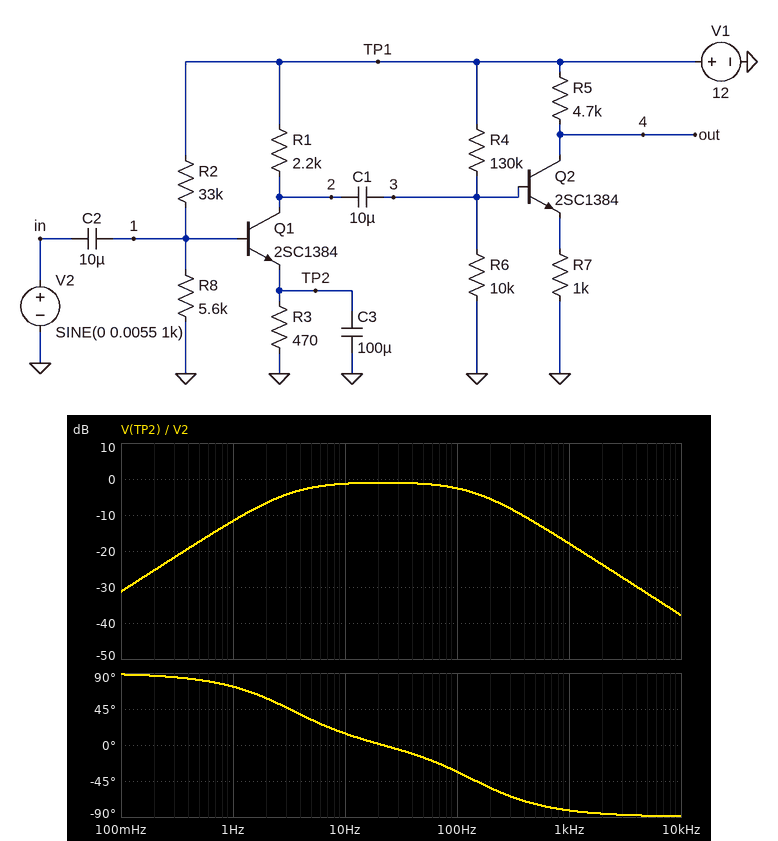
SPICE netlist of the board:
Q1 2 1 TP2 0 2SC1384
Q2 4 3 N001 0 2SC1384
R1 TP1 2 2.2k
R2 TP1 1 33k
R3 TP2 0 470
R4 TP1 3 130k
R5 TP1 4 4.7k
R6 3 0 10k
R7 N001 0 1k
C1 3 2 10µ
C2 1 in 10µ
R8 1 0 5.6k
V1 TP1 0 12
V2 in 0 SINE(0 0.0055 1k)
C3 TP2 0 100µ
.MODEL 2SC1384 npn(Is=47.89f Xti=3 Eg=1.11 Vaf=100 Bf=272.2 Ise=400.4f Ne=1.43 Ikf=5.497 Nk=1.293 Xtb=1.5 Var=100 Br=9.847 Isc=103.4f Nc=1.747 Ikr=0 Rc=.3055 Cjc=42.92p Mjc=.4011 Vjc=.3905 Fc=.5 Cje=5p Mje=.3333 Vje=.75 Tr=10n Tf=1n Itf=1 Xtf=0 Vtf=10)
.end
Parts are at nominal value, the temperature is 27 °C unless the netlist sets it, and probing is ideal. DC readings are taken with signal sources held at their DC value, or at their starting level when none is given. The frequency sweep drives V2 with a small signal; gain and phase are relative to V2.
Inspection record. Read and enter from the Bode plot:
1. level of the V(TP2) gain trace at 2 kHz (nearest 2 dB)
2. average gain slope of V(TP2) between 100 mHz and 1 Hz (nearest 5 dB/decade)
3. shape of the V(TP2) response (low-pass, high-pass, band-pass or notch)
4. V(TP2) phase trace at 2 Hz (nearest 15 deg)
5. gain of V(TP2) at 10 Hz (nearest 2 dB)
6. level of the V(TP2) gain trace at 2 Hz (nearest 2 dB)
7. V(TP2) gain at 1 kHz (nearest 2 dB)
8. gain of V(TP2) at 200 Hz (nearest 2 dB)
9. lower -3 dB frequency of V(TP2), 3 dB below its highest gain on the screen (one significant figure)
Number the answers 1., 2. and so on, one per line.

1. -24 dB
2. 20 dB/decade
3. band-pass
4. 60 deg
5. -2 dB
6. -6 dB
7. -18 dB
8. -6 dB
9. 3 Hz
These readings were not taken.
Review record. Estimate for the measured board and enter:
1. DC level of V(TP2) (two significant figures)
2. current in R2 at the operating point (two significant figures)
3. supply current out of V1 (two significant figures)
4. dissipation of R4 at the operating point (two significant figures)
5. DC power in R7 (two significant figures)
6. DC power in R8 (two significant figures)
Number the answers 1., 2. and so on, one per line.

1. 1.0 V
2. 310 µA
3. 2.8 mA
4. 960 µW
5. 63 µW
6. 490 µW
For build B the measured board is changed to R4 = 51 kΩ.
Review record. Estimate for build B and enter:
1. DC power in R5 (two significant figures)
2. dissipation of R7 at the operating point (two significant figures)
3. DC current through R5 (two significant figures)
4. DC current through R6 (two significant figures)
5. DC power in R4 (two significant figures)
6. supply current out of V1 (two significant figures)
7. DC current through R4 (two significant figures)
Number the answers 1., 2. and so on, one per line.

1. 7.2 mW
2. 1.6 mW
3. 1.2 mA
4. 190 µA
5. 2.0 mW
6. 3.9 mA
7. 200 µA
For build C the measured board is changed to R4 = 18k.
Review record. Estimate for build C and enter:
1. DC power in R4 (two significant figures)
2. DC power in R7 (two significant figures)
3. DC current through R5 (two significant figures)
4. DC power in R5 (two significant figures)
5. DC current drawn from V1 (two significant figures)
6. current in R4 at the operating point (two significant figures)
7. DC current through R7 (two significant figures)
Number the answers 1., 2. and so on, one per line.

1. 4.6 mW
2. 5.2 mW
3. 2.1 mA
4. 20 mW
5. 5.0 mA
6. 500 µA
7. 2.3 mA
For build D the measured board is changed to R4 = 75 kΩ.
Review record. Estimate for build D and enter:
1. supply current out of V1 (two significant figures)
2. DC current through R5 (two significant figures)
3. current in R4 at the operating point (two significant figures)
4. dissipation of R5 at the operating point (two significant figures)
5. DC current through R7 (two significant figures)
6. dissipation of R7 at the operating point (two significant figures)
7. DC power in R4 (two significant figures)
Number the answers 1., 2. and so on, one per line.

1. 3.3 mA
2. 730 µA
3. 140 µA
4. 2.5 mW
5. 740 µA
6. 550 µW
7. 1.5 mW
